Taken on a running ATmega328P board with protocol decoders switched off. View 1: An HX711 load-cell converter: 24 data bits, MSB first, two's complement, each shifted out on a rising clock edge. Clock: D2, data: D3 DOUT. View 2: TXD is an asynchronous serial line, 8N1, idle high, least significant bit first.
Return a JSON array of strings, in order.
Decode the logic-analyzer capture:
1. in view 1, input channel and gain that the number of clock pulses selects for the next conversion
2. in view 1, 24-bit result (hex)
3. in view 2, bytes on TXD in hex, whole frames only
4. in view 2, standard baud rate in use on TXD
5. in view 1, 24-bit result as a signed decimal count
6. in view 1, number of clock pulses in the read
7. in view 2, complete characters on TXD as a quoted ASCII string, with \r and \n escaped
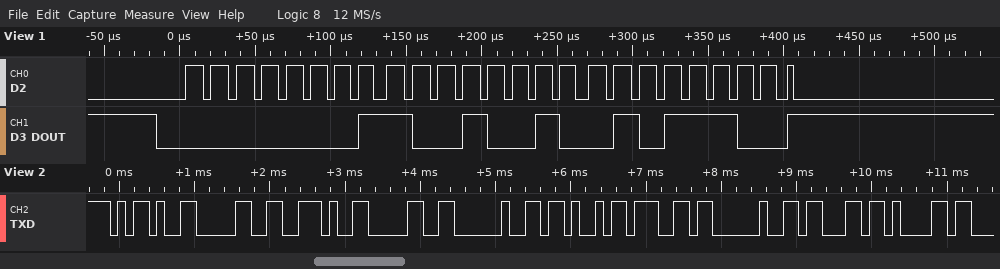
["channel A, gain 128", "0x01925C", "2D 30 2E 30 20 4B 67 20 63 61", "9600 baud", "103004", "25", "\"-0.0 Kg ca\""]
